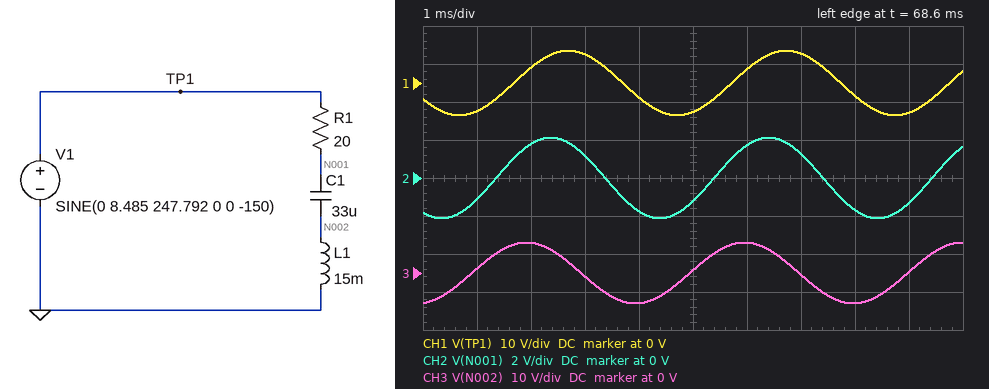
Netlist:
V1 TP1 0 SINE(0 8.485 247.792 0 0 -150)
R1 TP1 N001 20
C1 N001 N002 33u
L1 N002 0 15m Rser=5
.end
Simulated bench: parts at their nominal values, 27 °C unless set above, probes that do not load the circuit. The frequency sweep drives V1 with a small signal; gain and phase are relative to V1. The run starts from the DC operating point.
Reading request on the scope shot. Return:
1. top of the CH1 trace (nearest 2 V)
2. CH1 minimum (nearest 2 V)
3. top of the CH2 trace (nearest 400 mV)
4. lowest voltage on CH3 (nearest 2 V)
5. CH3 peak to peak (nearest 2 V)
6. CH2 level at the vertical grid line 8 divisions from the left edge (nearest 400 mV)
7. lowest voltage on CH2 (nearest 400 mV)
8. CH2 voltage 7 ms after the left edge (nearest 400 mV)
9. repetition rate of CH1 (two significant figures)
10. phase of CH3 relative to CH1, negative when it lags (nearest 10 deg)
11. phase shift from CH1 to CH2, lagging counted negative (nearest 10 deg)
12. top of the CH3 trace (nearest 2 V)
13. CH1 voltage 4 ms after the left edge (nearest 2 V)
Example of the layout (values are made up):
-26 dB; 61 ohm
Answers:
8 V; -8 V; 2.0 V; -8 V; 16 V; -1.6 V; -2.0 V; 1.2 V; 250 Hz; 70 deg; 30 deg; 8 V; -4 V
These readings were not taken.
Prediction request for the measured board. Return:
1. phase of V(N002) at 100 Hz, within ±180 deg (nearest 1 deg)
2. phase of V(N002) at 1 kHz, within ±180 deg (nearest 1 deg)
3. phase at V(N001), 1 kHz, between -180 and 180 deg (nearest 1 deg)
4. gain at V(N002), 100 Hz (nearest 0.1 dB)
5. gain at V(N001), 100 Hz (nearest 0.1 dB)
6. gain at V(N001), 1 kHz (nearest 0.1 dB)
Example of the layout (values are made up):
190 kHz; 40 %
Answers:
119 deg; 13 deg; 12 deg; -12.7 dB; -1.4 dB; -0.3 dB
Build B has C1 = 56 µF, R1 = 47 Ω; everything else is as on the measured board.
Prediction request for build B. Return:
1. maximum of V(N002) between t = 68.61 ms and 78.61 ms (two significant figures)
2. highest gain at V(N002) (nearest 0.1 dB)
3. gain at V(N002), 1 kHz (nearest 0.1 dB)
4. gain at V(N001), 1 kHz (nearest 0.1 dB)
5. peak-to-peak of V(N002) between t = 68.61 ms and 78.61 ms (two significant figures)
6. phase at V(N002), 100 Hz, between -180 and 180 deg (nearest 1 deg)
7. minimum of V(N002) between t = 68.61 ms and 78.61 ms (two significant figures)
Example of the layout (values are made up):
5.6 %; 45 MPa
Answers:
3.8 V; 0 dB; -0.9 dB; -1.2 dB; 7.6 V; 82 deg; -3.8 V
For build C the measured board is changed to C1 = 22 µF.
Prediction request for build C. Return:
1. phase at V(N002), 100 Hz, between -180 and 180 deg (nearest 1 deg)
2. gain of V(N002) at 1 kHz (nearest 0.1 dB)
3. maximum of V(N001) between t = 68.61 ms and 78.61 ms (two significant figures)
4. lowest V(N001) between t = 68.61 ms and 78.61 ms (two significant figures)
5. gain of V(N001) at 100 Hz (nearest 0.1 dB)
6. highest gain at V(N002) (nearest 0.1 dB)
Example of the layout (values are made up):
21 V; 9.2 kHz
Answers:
130 deg; 0.4 dB; 2.5 V; -2.5 V; -0.6 dB; 1.6 dB
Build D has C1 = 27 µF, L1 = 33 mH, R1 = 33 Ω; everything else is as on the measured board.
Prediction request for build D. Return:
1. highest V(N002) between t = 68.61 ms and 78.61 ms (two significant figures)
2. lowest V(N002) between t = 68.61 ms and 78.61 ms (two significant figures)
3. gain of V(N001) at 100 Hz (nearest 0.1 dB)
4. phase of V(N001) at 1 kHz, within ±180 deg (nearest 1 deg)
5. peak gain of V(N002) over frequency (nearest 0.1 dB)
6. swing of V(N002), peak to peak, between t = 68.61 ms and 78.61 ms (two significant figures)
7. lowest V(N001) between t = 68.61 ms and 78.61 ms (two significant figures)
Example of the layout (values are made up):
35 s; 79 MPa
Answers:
9.3 V; -9.3 V; -2.9 dB; 9 deg; 0.8 dB; 19 V; -5.1 V
